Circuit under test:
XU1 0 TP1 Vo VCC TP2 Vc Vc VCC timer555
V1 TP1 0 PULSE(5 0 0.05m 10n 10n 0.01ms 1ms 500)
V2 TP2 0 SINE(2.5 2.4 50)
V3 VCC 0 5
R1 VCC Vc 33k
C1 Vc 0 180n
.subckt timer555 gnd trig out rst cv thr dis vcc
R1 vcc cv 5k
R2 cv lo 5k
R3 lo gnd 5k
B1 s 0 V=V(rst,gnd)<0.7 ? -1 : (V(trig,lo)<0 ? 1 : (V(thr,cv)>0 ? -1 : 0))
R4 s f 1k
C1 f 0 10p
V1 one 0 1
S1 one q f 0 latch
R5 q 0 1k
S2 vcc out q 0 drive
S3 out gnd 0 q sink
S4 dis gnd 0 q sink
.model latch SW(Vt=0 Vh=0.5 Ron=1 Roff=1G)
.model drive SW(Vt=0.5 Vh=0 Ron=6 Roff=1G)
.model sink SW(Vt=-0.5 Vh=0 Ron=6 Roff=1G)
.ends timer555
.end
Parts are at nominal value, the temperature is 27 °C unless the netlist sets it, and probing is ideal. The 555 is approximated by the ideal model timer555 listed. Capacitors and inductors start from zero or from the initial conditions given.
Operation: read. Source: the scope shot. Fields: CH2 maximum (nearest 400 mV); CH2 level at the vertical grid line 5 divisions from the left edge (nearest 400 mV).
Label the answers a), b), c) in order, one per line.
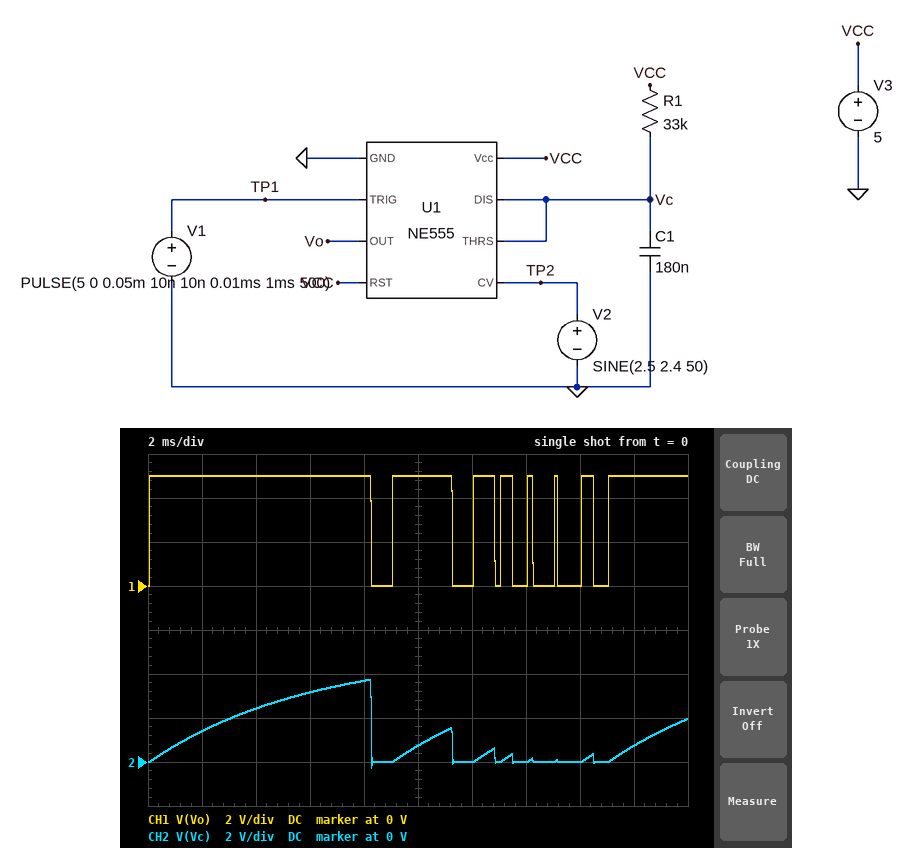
a) 3.6 V
b) 800 mV
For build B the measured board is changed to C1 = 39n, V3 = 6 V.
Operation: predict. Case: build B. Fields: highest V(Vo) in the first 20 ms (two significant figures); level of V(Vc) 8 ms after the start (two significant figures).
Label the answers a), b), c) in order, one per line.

a) 6.0 V
b) 3.1 V
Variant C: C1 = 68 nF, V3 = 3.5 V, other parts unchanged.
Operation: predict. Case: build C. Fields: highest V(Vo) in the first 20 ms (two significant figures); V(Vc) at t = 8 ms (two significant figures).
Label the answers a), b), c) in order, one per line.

a) 3.5 V
b) 3.4 V
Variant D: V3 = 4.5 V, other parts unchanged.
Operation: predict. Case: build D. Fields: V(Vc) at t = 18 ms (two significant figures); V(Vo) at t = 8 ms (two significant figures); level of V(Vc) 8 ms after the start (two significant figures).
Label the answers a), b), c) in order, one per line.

a) 670 mV
b) 4.5 V
c) 3.3 V
